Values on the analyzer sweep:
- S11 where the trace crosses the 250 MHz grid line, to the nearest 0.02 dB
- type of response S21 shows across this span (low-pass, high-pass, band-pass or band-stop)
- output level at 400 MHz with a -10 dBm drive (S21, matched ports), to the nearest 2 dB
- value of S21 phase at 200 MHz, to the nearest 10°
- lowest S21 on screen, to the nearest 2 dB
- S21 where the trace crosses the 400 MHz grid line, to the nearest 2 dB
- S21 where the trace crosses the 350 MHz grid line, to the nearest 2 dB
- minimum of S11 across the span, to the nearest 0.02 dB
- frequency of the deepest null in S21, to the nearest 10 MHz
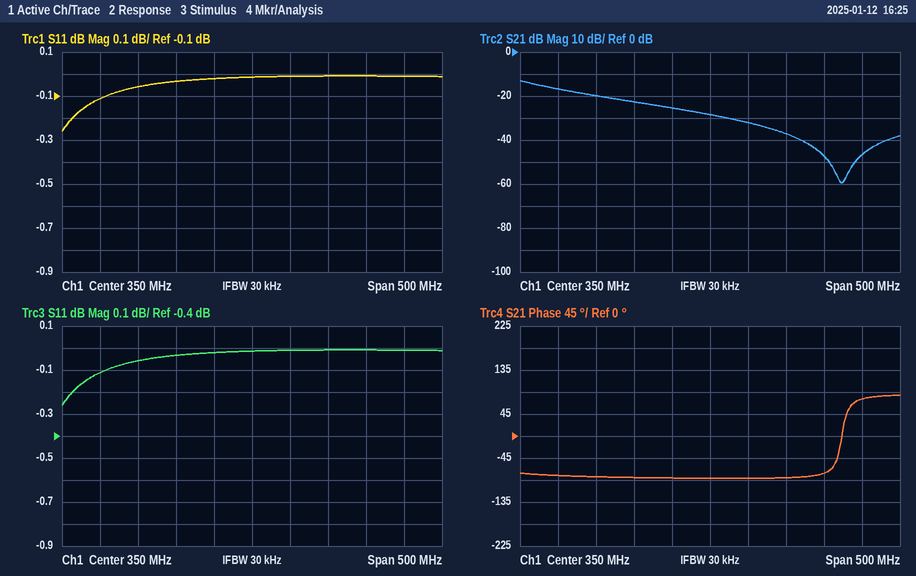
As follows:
-0.04 dB
low-pass
-42 dBm
-80°
-60 dB
-32 dB
-28 dB
-0.26 dB
520 MHz
